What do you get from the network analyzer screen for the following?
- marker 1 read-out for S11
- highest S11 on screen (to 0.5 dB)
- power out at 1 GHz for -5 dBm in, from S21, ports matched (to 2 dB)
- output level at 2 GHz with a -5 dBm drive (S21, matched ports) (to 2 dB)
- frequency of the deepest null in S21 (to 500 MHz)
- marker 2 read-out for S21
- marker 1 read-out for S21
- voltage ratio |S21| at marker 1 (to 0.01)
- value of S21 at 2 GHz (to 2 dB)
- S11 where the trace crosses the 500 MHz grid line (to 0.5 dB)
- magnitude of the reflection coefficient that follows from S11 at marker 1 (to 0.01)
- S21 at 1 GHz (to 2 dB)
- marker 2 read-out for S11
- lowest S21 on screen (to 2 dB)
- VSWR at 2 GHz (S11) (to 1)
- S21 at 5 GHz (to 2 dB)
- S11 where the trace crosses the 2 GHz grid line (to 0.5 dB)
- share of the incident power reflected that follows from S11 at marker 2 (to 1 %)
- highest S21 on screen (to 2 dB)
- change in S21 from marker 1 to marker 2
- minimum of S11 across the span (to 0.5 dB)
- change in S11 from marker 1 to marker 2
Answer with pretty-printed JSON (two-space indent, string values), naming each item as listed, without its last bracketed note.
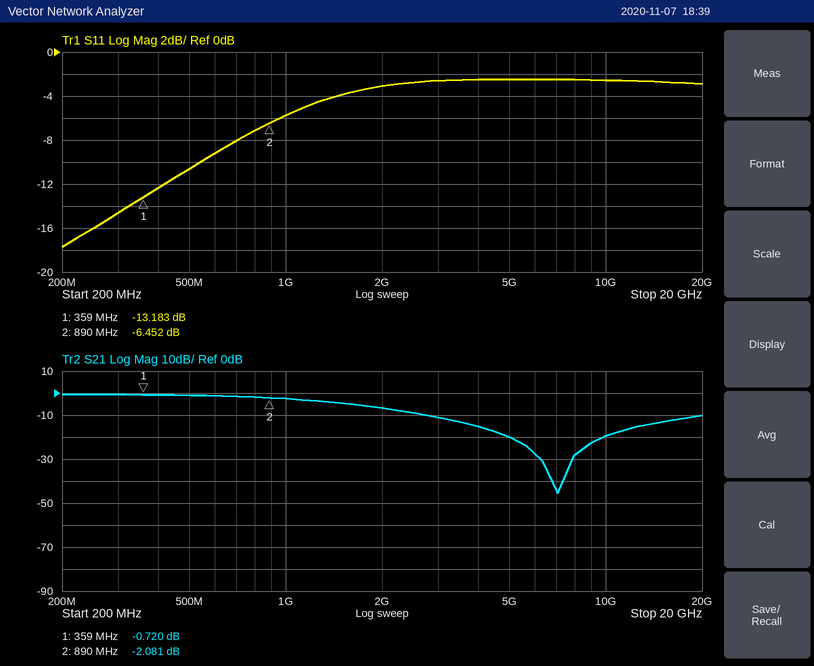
{
  "marker 1 read-out for S11": "-13.183 dB",
  "highest S11 on screen": "-2.5 dB",
  "power out at 1 GHz for -5 dBm in, from S21, ports matched": "-8 dBm",
  "output level at 2 GHz with a -5 dBm drive (S21, matched ports)": "-12 dBm",
  "frequency of the deepest null in S21": "7.0 GHz",
  "marker 2 read-out for S21": "-2.081 dB",
  "marker 1 read-out for S21": "-0.720 dB",
  "voltage ratio |S21| at marker 1": "0.92",
  "value of S21 at 2 GHz": "-6 dB",
  "S11 where the trace crosses the 500 MHz grid line": "-10.5 dB",
  "magnitude of the reflection coefficient that follows from S11 at marker 1": "0.22",
  "S21 at 1 GHz": "-2 dB",
  "marker 2 read-out for S11": "-6.452 dB",
  "lowest S21 on screen": "-46 dB",
  "VSWR at 2 GHz (S11)": "6",
  "S21 at 5 GHz": "-20 dB",
  "S11 where the trace crosses the 2 GHz grid line": "-3.0 dB",
  "share of the incident power reflected that follows from S11 at marker 2": "23 %",
  "highest S21 on screen": "0 dB",
  "change in S21 from marker 1 to marker 2": "-1.361 dB",
  "minimum of S11 across the span": "-17.5 dB",
  "change in S11 from marker 1 to marker 2": "6.731 dB"
}
